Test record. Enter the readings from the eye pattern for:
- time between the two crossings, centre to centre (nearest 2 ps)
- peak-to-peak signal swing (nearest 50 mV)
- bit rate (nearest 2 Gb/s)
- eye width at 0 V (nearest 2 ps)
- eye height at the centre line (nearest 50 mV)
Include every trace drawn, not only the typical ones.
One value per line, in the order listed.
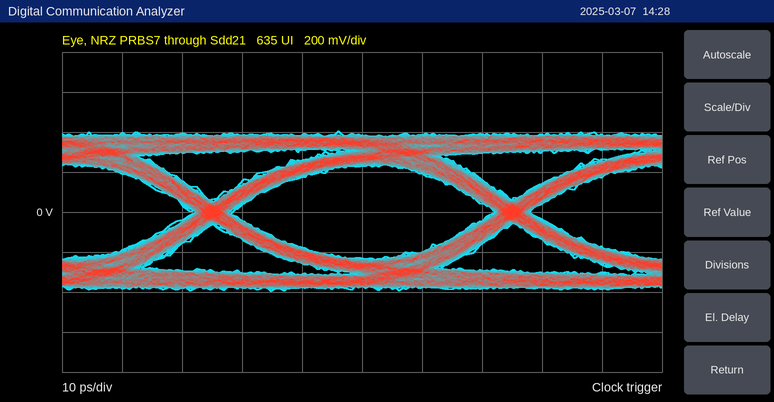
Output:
50 ps
800 mV
20 Gb/s
44 ps
450 mV
